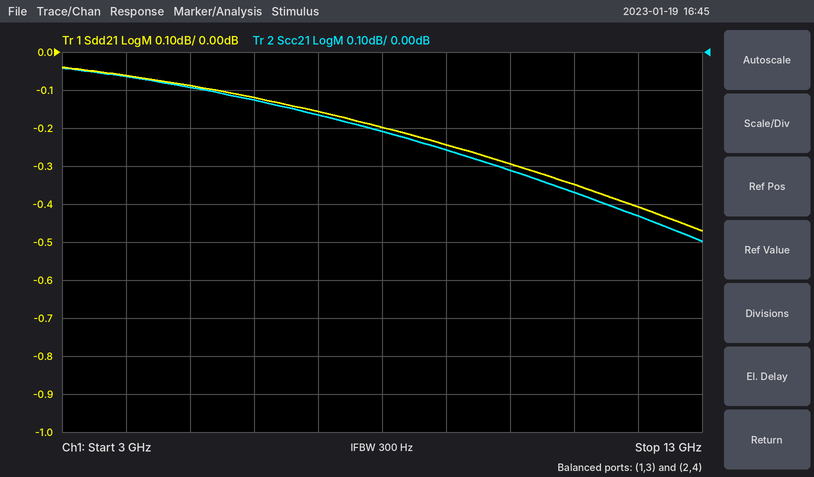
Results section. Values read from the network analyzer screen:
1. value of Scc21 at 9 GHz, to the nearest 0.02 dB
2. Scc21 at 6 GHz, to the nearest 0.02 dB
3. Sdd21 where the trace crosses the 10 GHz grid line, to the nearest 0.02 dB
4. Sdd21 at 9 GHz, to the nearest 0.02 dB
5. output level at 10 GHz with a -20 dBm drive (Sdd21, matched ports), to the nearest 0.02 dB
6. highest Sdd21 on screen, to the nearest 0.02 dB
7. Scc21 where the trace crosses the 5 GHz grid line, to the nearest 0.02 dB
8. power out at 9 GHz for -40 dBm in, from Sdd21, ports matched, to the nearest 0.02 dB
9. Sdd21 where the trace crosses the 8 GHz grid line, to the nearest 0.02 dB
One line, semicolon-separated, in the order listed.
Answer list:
-0.26 dB; -0.12 dB; -0.30 dB; -0.24 dB; -20.30 dBm; -0.04 dB; -0.10 dB; -40.24 dBm; -0.20 dB
